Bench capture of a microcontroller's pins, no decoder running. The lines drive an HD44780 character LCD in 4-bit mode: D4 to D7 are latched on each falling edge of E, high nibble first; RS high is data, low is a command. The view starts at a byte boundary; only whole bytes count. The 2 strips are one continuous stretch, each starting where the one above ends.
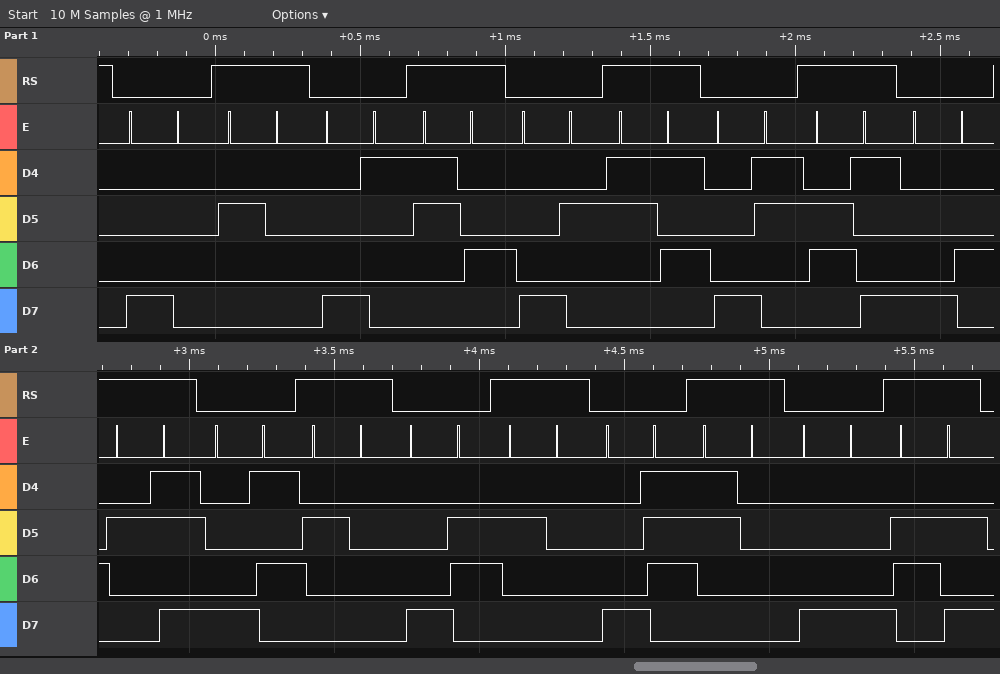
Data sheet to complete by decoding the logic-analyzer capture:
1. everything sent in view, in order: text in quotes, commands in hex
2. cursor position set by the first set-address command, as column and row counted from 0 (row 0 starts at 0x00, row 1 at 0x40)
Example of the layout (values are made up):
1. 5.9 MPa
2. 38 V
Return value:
1. 0x80 " " 0x81 "4" 0x82 "5" 0x83 "i" 0x84 "+" 0x85 " " 0x86 " " 0x87 "0" 0x88 "j"
2. column 0, row 0
